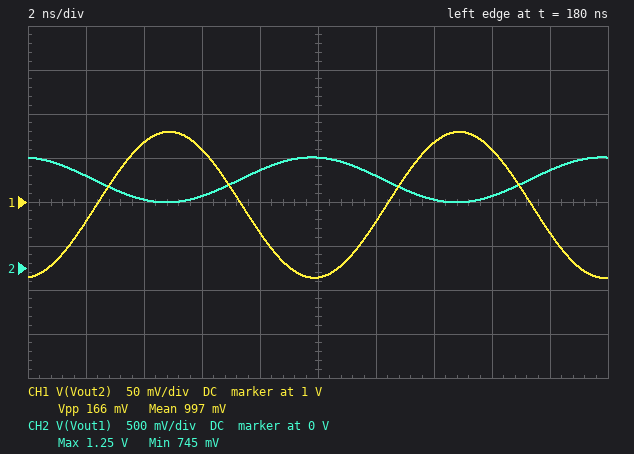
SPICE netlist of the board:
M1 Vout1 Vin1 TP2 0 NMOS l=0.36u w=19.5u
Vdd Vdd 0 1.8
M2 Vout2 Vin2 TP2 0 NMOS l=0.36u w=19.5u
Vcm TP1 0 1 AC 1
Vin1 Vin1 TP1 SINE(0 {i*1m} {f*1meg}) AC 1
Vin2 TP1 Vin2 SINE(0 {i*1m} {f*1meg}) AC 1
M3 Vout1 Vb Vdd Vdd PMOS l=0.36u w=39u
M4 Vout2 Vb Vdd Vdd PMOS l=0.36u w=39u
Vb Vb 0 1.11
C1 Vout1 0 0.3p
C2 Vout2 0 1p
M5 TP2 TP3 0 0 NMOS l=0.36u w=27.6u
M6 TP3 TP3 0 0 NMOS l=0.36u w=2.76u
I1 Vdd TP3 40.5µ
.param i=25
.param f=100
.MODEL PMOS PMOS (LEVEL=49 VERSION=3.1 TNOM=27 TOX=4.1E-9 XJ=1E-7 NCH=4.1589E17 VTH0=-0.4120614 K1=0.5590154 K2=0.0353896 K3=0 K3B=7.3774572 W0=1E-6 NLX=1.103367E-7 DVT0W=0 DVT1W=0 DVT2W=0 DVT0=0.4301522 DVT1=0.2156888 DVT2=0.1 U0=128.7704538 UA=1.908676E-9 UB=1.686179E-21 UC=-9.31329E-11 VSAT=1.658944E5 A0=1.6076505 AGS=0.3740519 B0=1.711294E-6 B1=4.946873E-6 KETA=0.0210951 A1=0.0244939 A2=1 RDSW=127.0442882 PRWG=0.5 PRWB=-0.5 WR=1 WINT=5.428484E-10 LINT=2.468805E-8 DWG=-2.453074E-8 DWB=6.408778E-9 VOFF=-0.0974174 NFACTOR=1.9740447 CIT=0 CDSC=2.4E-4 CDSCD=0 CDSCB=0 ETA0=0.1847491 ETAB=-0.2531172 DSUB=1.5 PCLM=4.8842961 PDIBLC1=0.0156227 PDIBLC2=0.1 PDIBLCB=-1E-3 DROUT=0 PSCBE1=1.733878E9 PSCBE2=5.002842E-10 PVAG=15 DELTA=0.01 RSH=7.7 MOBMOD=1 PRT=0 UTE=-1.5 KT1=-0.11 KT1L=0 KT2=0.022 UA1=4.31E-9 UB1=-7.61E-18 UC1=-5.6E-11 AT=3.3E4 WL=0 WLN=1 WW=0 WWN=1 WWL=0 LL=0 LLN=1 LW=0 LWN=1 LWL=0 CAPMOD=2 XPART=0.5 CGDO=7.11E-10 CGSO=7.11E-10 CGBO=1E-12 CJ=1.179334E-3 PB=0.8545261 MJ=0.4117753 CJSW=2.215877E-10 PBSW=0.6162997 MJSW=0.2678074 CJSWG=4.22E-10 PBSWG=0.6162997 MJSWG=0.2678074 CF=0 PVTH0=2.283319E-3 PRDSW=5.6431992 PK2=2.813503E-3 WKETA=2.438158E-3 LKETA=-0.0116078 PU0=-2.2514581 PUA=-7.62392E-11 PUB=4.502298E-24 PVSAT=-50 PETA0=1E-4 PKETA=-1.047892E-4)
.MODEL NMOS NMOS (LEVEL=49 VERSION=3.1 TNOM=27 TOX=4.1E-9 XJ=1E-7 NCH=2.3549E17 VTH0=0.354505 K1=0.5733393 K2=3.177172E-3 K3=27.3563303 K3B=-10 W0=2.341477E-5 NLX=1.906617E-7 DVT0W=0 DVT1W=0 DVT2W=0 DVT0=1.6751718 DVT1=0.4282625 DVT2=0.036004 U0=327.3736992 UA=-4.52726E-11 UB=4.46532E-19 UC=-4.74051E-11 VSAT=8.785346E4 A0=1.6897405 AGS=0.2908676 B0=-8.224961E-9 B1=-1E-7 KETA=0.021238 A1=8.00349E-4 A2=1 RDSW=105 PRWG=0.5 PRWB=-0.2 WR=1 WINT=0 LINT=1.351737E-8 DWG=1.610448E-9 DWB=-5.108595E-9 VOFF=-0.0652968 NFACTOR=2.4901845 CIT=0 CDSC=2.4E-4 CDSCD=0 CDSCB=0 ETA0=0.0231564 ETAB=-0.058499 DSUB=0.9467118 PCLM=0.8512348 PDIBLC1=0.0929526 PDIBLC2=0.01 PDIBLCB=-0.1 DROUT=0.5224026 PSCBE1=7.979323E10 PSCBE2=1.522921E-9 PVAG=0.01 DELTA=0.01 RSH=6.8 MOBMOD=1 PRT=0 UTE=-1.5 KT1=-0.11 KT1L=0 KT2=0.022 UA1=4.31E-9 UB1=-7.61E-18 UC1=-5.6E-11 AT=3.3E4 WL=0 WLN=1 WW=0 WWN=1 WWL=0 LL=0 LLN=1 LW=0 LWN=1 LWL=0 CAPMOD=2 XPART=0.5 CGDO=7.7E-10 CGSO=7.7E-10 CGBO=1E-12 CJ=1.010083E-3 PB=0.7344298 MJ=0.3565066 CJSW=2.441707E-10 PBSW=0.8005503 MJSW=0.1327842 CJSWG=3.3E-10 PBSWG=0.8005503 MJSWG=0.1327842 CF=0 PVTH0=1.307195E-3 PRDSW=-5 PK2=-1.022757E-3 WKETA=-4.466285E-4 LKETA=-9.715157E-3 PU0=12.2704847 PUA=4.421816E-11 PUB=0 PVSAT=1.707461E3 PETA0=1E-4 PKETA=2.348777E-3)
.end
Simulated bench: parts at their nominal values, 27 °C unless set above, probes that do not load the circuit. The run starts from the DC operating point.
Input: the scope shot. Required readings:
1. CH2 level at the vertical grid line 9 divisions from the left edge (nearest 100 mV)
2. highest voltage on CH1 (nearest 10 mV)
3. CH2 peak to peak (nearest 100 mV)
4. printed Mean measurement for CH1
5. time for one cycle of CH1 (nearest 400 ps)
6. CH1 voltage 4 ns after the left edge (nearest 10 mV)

1.1 V
1.08 V
500 mV
997 mV
10.0 ns
1.07 V
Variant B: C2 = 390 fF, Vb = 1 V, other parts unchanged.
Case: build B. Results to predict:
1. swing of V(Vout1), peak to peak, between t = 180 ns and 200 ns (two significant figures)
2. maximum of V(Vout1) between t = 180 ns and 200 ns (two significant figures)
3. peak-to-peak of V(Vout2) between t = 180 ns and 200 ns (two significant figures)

64 mV
1.7 V
63 mV
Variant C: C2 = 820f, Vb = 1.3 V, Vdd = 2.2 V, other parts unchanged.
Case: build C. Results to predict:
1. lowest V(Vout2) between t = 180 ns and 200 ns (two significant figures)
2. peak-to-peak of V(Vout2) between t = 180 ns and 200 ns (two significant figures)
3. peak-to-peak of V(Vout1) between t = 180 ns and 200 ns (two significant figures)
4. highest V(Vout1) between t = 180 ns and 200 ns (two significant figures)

2.1 V
41 mV
42 mV
2.2 V
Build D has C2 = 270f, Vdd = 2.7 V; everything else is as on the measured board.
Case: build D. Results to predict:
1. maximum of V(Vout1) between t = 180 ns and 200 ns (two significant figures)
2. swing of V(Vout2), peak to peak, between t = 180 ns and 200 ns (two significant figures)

2.7 V
18 mV
